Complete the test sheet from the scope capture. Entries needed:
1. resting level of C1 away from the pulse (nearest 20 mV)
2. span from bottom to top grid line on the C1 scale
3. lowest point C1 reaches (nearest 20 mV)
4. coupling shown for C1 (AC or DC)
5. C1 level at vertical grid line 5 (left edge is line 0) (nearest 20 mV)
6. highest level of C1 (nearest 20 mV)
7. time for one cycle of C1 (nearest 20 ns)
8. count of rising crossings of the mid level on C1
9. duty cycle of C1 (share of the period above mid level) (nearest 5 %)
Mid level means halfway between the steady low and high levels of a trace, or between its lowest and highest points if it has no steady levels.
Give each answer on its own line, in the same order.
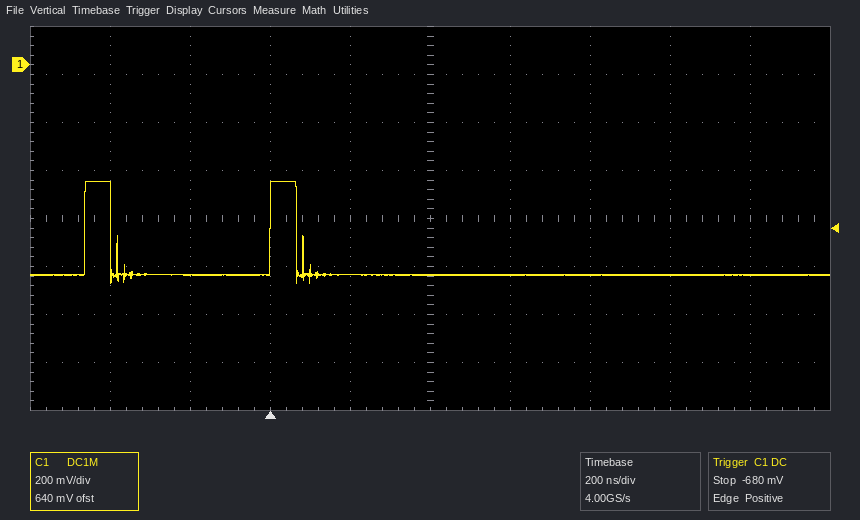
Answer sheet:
-880 mV
1.6 V
-920 mV
DC
-880 mV
-480 mV
460 ns
2
15 %
